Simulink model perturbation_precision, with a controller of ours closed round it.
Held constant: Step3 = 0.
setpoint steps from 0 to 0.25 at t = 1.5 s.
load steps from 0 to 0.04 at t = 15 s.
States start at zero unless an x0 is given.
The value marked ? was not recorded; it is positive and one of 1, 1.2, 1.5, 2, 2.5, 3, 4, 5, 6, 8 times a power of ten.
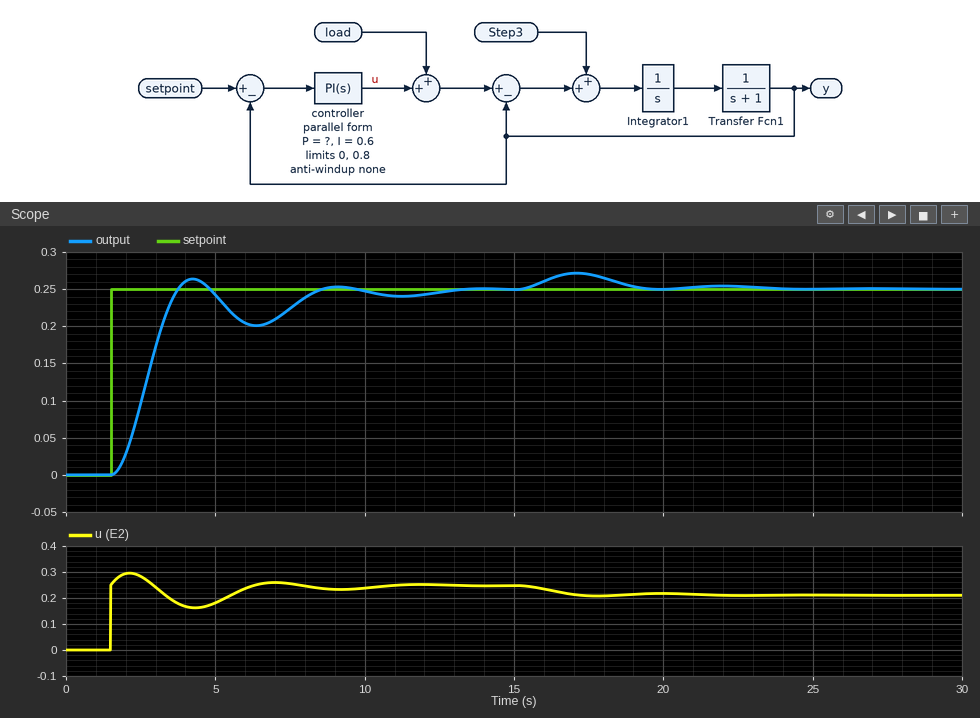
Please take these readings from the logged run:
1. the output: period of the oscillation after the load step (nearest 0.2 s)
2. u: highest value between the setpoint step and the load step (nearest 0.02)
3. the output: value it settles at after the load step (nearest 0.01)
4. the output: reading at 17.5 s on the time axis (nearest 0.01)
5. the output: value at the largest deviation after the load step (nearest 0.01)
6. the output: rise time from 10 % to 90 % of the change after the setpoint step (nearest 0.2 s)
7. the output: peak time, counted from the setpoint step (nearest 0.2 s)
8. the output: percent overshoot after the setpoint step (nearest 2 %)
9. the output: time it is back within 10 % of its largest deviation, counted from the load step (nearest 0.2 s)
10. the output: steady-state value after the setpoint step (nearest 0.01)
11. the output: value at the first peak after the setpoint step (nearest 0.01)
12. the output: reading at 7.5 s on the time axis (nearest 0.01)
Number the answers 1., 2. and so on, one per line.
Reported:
1. 4.8 s
2. 0.30
3. 0.25
4. 0.27
5. 0.27
6. 1.4 s
7. 2.8 s
8. 6 %
9. 8.2 s
10. 0.25
11. 0.26
12. 0.22
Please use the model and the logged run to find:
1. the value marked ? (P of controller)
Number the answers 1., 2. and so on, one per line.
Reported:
1. 1
